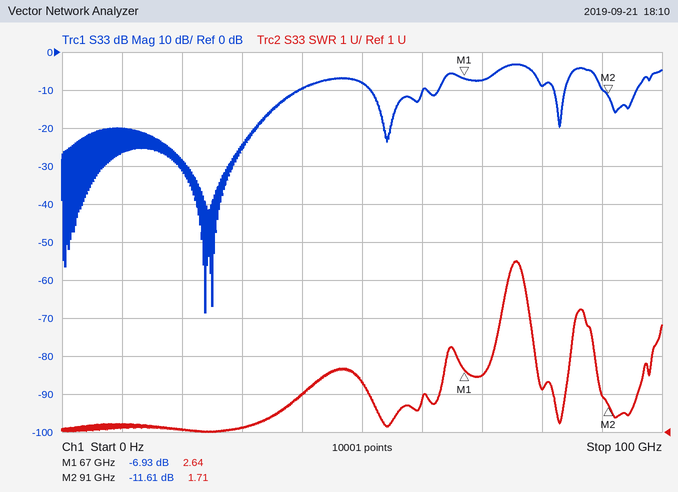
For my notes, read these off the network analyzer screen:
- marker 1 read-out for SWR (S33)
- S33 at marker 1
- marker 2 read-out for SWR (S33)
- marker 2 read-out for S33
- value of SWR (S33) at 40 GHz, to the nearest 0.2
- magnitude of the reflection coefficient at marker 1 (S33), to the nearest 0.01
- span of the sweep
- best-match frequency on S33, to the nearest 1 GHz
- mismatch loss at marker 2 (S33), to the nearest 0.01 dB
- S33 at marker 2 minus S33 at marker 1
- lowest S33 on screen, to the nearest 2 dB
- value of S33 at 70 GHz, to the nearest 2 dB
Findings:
2.64
-6.93 dB
1.71
-11.61 dB
2.0
0.45
100 GHz
24 GHz
0.31 dB
-4.68 dB
-68 dB
-8 dB
